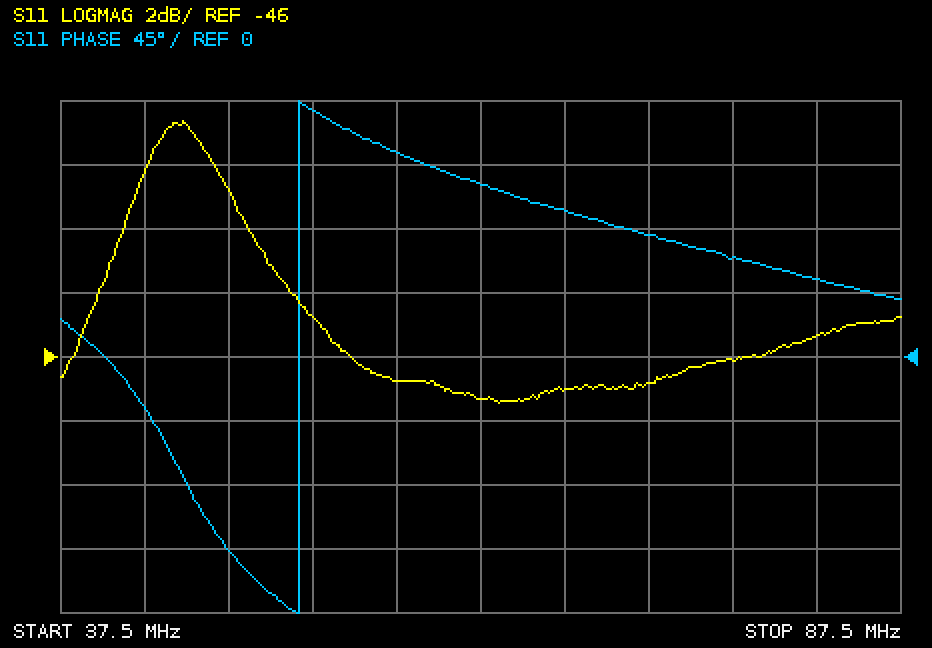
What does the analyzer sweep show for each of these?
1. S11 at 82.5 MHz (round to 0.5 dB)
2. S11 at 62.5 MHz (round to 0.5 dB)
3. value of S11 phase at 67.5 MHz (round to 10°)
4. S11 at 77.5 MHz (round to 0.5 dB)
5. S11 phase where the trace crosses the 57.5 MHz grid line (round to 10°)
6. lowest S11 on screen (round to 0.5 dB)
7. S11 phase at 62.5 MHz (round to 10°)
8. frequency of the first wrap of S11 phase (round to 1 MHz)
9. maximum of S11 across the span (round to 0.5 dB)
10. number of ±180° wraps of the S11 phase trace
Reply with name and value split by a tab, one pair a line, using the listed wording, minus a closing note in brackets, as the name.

S11 at 82.5 MHz	-45.5 dB
S11 at 62.5 MHz	-47.5 dB
value of S11 phase at 67.5 MHz	100°
S11 at 77.5 MHz	-46.0 dB
S11 phase where the trace crosses the 57.5 MHz grid line	140°
lowest S11 on screen	-47.5 dB
S11 phase at 62.5 MHz	120°
frequency of the first wrap of S11 phase	52 MHz
maximum of S11 across the span	-38.5 dB
number of ±180° wraps of the S11 phase trace	1
